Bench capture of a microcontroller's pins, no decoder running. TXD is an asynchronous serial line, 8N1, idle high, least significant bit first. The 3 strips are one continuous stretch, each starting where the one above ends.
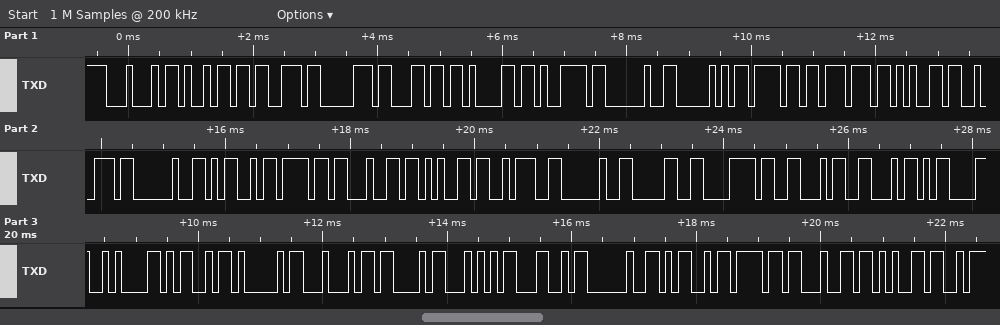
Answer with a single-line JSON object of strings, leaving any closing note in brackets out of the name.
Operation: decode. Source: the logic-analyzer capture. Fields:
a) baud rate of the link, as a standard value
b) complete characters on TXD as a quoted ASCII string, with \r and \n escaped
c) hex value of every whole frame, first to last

{"baud rate of the link, as a standard value": "9600 baud", "complete characters on TXD as a quoted ASCII string, with \\r and \\n escaped": "\"Display Power Mode: 0xFF\\r\\nMADCTL Mode\"", "hex value of every whole frame, first to last": "44 69 73 70 6C 61 79 20 50 6F 77 65 72 20 4D 6F 64 65 3A 20 30 78 46 46 0D 0A 4D 41 44 43 54 4C 20 4D 6F 64 65"}
